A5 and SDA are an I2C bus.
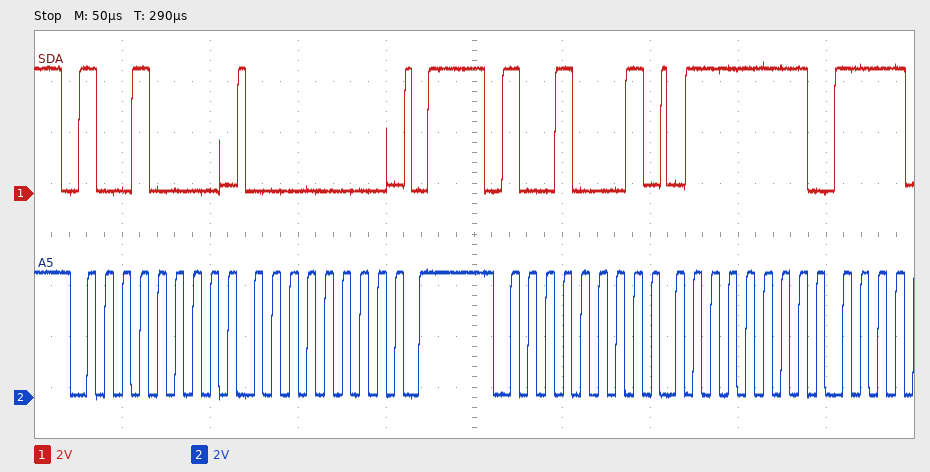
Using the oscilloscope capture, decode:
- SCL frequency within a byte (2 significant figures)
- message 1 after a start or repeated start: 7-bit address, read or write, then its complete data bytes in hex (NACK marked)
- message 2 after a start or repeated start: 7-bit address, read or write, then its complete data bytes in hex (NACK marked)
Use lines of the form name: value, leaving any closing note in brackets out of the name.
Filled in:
SCL frequency within a byte: 100 kHz
message 1 after a start or repeated start: 7-bit address, read or write, then its complete data bytes in hex: 0x48 write: 00
message 2 after a start or repeated start: 7-bit address, read or write, then its complete data bytes in hex: 0x48 read: 7F
